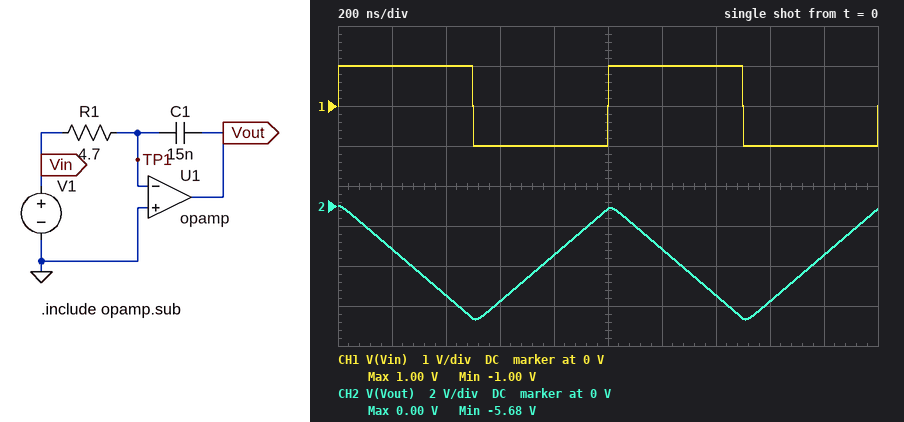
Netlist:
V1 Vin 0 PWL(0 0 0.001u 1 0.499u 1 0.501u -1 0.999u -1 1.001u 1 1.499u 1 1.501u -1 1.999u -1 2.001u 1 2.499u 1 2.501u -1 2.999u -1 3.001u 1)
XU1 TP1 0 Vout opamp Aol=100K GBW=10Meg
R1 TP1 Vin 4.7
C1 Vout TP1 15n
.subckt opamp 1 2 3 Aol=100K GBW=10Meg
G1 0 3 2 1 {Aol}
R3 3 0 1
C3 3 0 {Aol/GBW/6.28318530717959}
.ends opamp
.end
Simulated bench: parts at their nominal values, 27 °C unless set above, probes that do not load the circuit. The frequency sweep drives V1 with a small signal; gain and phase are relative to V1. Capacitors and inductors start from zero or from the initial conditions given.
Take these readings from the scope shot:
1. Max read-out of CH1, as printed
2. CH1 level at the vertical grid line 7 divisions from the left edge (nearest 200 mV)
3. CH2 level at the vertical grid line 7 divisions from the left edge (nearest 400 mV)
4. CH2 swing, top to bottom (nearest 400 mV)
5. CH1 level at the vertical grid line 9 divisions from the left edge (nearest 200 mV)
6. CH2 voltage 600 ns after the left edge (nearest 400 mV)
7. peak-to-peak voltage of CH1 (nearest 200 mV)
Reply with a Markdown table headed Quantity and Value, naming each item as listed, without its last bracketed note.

| Quantity | Value |
|---|---|
| Max read-out of CH1, as printed | 1.00 V |
| CH1 level at the vertical grid line 7 divisions from the left edge | 1.0 V |
| CH2 level at the vertical grid line 7 divisions from the left edge | -4.4 V |
| CH2 swing, top to bottom | 5.6 V |
| CH1 level at the vertical grid line 9 divisions from the left edge | -1.0 V |
| CH2 voltage 600 ns after the left edge | -4.8 V |
| peak-to-peak voltage of CH1 | 2.0 V |
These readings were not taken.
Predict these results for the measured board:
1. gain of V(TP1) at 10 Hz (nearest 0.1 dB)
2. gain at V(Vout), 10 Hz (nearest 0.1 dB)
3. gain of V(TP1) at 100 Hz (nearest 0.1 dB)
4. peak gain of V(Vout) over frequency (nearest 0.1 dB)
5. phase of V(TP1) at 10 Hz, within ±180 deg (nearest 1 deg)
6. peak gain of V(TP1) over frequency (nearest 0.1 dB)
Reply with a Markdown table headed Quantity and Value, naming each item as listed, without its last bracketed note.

| Quantity | Value |
|---|---|
| gain of V(TP1) at 10 Hz | -1.1 dB |
| gain at V(Vout), 10 Hz | 98.9 dB |
| gain of V(TP1) at 100 Hz | -11.8 dB |
| peak gain of V(Vout) over frequency | 100.0 dB |
| phase of V(TP1) at 10 Hz, within ±180 deg | -23 deg |
| peak gain of V(TP1) over frequency | 0 dB |
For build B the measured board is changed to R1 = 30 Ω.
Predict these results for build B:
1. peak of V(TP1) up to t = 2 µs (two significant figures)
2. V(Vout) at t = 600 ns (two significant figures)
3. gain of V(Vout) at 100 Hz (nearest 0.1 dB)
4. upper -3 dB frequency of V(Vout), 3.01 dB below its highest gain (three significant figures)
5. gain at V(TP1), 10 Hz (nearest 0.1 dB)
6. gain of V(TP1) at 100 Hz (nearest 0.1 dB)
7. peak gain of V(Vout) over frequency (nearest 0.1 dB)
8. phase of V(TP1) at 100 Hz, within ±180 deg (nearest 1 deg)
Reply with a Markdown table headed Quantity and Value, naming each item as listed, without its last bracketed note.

| Quantity | Value |
|---|---|
| peak of V(TP1) up to t = 2 µs | 34 mV |
| V(Vout) at t = 600 ns | -890 mV |
| gain of V(Vout) at 100 Hz | 70.7 dB |
| upper -3 dB frequency of V(Vout), 3.01 dB below its highest gain | 3.42 Hz |
| gain at V(TP1), 10 Hz | -9.8 dB |
| gain of V(TP1) at 100 Hz | -26.3 dB |
| peak gain of V(Vout) over frequency | 100.0 dB |
| phase of V(TP1) at 100 Hz, within ±180 deg | -43 deg |
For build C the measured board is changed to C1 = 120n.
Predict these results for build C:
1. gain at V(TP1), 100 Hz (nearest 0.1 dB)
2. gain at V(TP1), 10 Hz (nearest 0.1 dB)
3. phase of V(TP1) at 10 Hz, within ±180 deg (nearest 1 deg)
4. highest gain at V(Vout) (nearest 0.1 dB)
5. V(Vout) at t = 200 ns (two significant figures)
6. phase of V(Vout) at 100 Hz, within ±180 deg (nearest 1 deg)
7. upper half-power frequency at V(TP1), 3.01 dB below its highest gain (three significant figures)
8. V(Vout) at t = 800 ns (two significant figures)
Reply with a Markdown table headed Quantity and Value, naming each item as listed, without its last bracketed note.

| Quantity | Value |
|---|---|
| gain at V(TP1), 100 Hz | -28.2 dB |
| gain at V(TP1), 10 Hz | -11.5 dB |
| phase of V(TP1) at 10 Hz, within ±180 deg | -69 deg |
| highest gain at V(Vout) | 100.0 dB |
| V(Vout) at t = 200 ns | -320 mV |
| phase of V(Vout) at 100 Hz, within ±180 deg | 92 deg |
| upper half-power frequency at V(TP1), 3.01 dB below its highest gain | 2.75 Hz |
| V(Vout) at t = 800 ns | -370 mV |
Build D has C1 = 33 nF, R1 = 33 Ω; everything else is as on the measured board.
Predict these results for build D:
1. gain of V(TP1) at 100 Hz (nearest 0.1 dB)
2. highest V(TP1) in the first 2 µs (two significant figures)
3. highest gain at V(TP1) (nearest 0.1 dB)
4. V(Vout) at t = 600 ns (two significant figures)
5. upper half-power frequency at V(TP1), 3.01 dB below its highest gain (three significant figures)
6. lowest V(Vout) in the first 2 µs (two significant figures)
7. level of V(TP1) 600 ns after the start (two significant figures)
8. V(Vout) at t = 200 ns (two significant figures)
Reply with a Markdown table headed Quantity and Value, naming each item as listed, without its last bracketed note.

| Quantity | Value |
|---|---|
| gain of V(TP1) at 100 Hz | -33.8 dB |
| highest V(TP1) in the first 2 µs | 14 mV |
| highest gain at V(TP1) | 0 dB |
| V(Vout) at t = 600 ns | -380 mV |
| upper half-power frequency at V(TP1), 3.01 dB below its highest gain | 1.44 Hz |
| lowest V(Vout) in the first 2 µs | -440 mV |
| level of V(TP1) 600 ns after the start | -14 mV |
| V(Vout) at t = 200 ns | -170 mV |
